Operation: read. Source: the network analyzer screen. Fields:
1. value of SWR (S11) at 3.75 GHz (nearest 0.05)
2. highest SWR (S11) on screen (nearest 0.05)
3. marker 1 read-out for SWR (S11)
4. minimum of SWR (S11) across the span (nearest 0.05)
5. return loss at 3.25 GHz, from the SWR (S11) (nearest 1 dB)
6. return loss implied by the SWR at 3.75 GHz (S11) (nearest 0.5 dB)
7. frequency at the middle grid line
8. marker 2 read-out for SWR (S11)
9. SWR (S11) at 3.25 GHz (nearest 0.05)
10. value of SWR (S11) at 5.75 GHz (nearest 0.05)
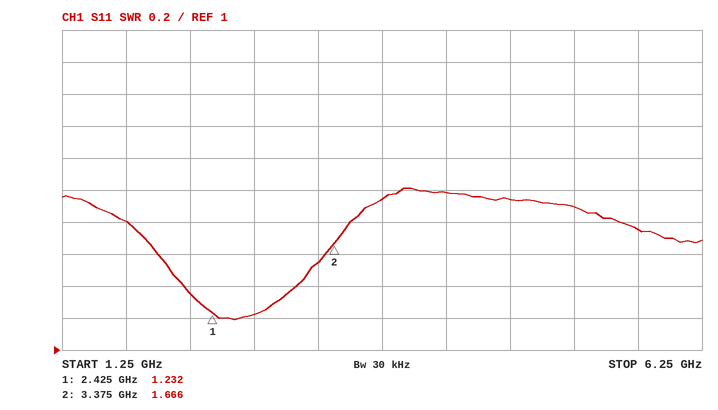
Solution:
1.95
2.00
1.232
1.20
13 dB
10.0 dB
3.75 GHz
1.666
1.55
1.75
